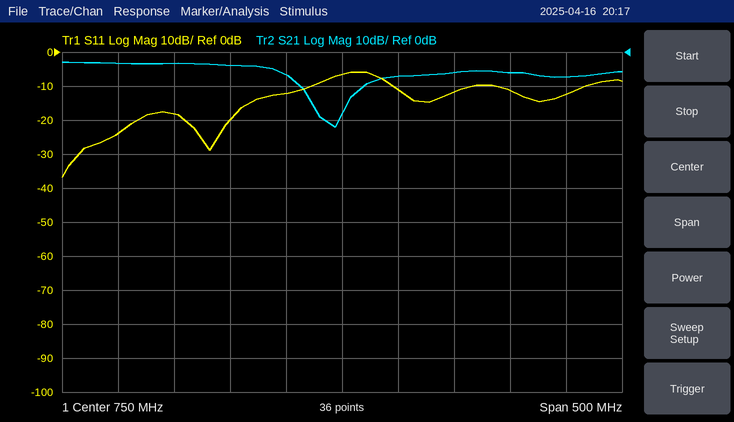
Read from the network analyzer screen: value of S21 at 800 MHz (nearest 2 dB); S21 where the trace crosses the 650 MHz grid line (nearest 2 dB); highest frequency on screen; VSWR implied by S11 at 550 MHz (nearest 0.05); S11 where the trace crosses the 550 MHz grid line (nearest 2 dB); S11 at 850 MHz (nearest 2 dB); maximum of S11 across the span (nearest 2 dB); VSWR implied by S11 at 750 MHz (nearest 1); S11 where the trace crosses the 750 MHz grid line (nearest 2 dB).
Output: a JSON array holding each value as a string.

["-8 dB", "-4 dB", "1 GHz", "1.15", "-24 dB", "-12 dB", "-6 dB", "3", "-6 dB"]
